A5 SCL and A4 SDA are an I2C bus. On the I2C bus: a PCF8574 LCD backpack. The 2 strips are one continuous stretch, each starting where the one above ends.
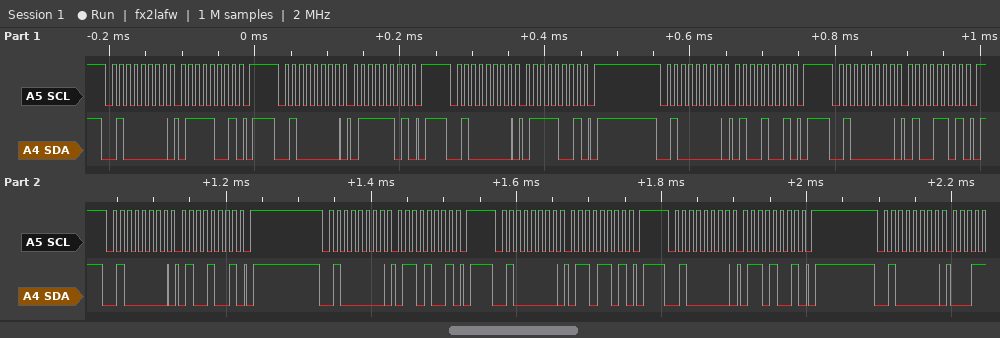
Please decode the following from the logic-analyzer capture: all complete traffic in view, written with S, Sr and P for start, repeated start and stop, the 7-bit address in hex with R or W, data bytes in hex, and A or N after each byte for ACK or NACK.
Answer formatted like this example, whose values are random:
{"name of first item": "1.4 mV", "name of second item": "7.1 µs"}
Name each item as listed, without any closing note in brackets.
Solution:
{"all complete traffic in view, written with S, Sr and P for start, repeated start and stop, the 7-bit address in hex with R or W, data bytes in hex, and A or N after each byte for ACK or NACK": "S 20W A 79 A P S 20W A 7D A P S 20W A 79 A P S 20W A 49 A P S 20W A 4D A P S 20W A 49 A P S 20W A 69 A P S 20W A 6D A P S 20W A 69 A P S 20W A"}
